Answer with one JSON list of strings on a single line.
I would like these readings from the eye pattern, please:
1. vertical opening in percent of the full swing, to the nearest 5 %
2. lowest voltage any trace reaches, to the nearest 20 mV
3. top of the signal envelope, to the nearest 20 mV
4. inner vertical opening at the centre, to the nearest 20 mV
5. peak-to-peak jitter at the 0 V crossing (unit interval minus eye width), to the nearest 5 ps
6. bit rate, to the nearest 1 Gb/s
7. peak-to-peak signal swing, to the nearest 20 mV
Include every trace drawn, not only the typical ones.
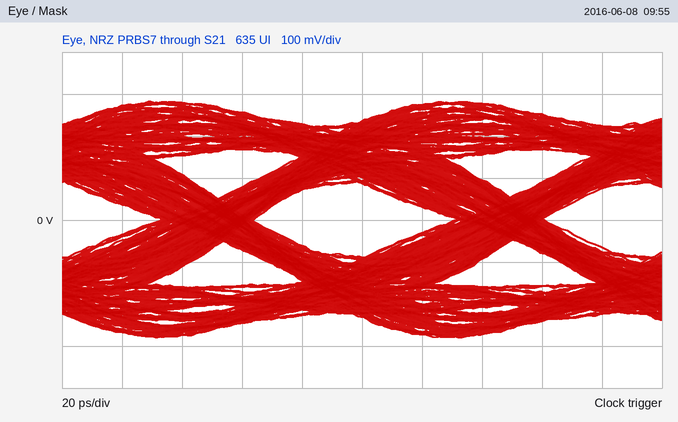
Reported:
["30 %", "-280 mV", "280 mV", "180 mV", "30 ps", "10 Gb/s", "560 mV"]
